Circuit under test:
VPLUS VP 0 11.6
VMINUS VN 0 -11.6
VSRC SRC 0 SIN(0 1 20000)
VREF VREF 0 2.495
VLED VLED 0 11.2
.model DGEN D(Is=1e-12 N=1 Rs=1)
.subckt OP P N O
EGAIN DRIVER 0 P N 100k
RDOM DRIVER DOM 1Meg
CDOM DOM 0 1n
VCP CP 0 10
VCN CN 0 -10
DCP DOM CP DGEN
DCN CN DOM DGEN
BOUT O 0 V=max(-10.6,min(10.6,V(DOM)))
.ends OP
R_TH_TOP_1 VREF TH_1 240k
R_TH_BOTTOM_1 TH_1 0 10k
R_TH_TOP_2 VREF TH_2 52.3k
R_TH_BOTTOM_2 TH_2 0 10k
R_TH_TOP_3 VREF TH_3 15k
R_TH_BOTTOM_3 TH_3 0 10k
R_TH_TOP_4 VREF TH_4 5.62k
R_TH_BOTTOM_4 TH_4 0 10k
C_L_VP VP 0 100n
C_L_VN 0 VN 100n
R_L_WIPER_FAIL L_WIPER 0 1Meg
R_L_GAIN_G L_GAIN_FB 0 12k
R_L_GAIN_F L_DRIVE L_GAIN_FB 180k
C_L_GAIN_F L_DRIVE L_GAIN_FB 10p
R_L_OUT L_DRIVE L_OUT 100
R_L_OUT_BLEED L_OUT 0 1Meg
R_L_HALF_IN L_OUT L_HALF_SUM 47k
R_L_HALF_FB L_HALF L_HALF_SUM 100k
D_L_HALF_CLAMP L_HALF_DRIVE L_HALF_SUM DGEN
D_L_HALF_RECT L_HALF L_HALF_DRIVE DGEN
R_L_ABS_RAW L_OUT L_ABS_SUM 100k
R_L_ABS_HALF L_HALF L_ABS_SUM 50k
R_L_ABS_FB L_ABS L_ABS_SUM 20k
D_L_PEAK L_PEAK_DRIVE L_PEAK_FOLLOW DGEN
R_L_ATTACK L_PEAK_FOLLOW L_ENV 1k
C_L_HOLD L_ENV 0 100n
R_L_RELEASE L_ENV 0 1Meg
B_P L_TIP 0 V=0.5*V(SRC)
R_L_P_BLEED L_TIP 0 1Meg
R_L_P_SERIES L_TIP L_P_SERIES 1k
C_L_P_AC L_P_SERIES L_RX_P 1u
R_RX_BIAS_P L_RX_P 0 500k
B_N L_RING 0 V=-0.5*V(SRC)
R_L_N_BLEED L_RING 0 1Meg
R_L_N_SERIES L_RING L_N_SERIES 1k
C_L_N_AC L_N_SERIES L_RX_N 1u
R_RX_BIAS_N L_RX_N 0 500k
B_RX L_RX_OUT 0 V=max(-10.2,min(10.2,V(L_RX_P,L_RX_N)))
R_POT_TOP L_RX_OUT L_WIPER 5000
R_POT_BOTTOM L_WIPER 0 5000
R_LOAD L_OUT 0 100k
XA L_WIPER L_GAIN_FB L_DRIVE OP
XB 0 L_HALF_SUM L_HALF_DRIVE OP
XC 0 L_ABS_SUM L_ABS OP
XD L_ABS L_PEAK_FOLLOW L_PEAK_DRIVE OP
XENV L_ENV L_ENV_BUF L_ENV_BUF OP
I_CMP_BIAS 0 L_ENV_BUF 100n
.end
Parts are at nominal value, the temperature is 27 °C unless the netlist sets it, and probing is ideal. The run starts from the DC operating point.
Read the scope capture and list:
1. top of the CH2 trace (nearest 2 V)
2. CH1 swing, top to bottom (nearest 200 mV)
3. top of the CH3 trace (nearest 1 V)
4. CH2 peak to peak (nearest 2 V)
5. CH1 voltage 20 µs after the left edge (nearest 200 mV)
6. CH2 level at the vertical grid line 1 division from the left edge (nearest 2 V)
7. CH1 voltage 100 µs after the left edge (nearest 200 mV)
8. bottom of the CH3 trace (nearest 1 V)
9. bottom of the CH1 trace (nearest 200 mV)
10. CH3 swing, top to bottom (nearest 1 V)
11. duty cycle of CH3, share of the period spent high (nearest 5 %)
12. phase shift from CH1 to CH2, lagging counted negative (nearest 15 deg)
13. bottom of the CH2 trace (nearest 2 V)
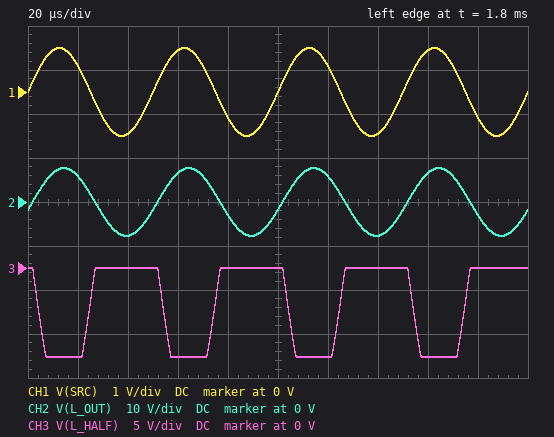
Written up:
8 V
2.0 V
0 V
16 V
600 mV
6 V
0 V
-10 V
-1.0 V
10 V
60 %
-15 deg
-8 V
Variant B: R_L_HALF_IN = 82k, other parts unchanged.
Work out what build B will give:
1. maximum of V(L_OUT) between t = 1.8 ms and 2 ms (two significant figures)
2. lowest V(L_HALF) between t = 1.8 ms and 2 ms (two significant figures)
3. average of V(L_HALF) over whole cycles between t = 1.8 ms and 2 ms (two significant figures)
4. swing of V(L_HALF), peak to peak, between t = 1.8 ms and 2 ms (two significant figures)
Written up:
7.7 V
-9.4 V
-3.0 V
9.4 V
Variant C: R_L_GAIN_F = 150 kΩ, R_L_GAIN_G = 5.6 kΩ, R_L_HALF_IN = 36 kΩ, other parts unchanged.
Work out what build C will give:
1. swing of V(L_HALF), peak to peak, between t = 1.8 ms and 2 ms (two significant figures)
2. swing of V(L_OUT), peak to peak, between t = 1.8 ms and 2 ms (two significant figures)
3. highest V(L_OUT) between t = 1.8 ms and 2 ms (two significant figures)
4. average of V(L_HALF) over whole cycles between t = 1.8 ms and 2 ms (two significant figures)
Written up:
10 V
21 V
11 V
-4.6 V
